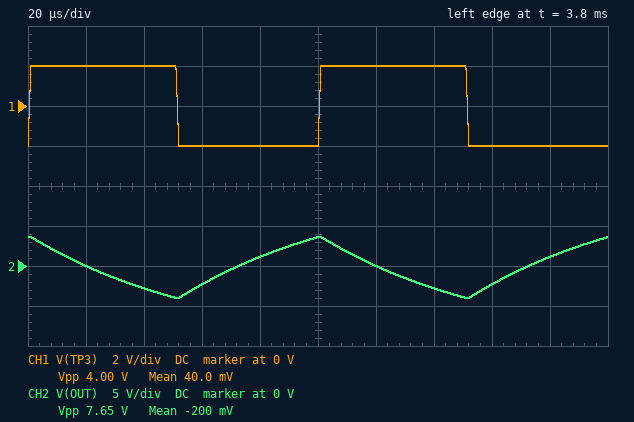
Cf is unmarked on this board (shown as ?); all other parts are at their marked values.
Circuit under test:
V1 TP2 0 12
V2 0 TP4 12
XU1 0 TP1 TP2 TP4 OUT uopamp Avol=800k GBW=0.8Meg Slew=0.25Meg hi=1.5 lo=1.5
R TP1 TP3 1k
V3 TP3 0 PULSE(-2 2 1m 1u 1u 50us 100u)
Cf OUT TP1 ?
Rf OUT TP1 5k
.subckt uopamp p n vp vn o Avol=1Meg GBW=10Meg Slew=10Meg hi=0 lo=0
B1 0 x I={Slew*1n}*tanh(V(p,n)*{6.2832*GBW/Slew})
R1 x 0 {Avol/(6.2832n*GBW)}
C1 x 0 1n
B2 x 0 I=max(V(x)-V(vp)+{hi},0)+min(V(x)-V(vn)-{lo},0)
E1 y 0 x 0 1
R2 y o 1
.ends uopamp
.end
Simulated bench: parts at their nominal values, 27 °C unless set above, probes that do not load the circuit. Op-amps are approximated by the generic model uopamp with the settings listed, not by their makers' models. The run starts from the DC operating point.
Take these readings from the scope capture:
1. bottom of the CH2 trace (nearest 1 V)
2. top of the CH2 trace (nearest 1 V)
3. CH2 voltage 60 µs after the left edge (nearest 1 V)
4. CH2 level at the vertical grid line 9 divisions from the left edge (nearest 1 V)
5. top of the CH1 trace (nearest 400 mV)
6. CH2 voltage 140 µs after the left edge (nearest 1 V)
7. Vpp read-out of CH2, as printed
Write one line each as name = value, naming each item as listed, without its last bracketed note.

bottom of the CH2 trace = -4 V
top of the CH2 trace = 4 V
CH2 voltage 60 µs after the left edge = -2 V
CH2 level at the vertical grid line 9 divisions from the left edge = 1 V
top of the CH1 trace = 2.0 V
CH2 voltage 140 µs after the left edge = -3 V
Vpp read-out of CH2, as printed = 7.65 V
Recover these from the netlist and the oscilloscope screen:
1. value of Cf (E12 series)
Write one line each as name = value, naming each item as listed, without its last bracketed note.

value of Cf = 12 nF
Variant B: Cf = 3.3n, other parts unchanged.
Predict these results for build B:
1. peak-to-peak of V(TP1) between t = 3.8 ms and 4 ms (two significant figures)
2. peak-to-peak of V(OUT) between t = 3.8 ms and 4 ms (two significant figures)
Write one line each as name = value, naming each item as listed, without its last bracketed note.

peak-to-peak of V(TP1) between t = 3.8 ms and 4 ms = 3.3 V
peak-to-peak of V(OUT) between t = 3.8 ms and 4 ms = 12 V
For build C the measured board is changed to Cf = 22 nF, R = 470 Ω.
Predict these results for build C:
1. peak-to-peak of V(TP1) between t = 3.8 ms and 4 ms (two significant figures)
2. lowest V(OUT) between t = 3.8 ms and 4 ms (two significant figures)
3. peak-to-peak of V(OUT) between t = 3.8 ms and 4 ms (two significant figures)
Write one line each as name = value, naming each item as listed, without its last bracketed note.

peak-to-peak of V(TP1) between t = 3.8 ms and 4 ms = 140 mV
lowest V(OUT) between t = 3.8 ms and 4 ms = -5.0 V
peak-to-peak of V(OUT) between t = 3.8 ms and 4 ms = 9.2 V
